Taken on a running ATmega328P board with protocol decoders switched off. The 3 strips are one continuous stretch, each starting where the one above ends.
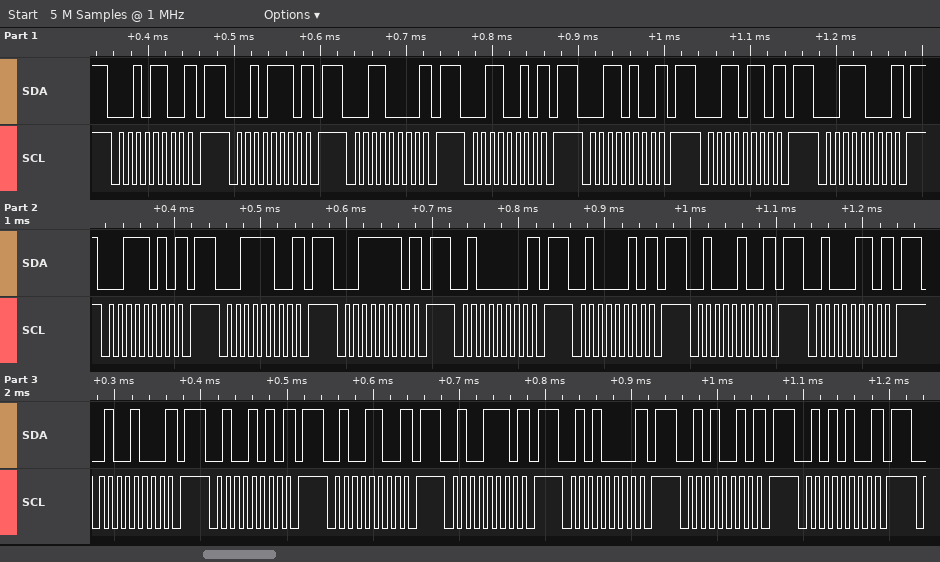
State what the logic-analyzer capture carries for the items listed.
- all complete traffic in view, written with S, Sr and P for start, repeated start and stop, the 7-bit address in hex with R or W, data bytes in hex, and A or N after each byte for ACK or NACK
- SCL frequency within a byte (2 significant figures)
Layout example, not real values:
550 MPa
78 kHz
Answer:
S 16W N P S 17W N P S 18W N P S 19W N P S 1AW N P S 1BW N P S 1CW N P S 1DW N P S 1EW N P S 1FW N P S 20W N P S 21W N P S 22W N P S 23W N P S 24W N P S 25W N P S 26W N P S 27W N P S 28W N P S 29W N P S 2AW N P
100 kHz
